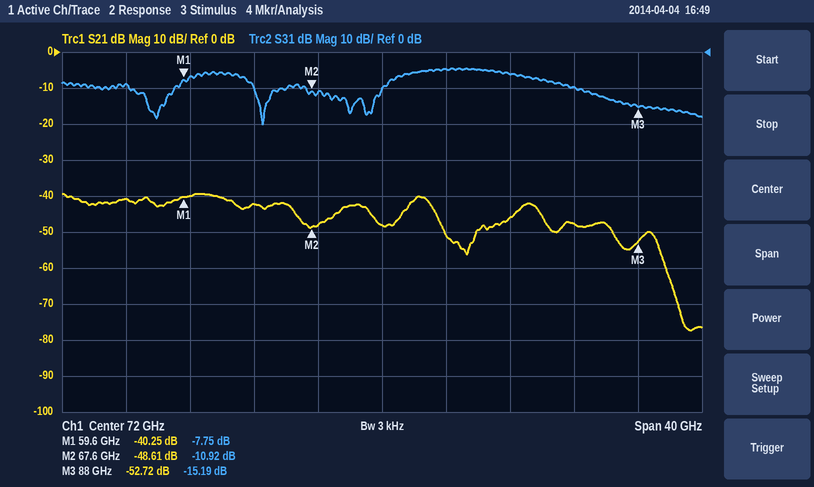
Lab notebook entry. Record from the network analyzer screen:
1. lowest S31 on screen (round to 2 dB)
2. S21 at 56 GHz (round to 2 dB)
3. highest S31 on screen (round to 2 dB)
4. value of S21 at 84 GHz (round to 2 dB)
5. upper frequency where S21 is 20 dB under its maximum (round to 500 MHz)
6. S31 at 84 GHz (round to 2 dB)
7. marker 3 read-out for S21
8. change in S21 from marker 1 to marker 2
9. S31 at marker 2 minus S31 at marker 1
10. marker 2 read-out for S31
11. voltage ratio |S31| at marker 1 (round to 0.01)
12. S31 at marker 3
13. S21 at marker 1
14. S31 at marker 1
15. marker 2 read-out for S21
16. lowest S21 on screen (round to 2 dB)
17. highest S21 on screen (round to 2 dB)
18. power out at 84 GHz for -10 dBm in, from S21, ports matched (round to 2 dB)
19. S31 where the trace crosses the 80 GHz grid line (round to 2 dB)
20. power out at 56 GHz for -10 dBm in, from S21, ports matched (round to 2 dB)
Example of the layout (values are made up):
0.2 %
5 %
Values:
-20 dB
-40 dB
-4 dB
-48 dB
89.5 GHz
-10 dB
-52.72 dB
-8.36 dB
-3.17 dB
-10.92 dB
0.41
-15.19 dB
-40.25 dB
-7.75 dB
-48.61 dB
-78 dB
-40 dB
-58 dBm
-6 dB
-50 dBm
